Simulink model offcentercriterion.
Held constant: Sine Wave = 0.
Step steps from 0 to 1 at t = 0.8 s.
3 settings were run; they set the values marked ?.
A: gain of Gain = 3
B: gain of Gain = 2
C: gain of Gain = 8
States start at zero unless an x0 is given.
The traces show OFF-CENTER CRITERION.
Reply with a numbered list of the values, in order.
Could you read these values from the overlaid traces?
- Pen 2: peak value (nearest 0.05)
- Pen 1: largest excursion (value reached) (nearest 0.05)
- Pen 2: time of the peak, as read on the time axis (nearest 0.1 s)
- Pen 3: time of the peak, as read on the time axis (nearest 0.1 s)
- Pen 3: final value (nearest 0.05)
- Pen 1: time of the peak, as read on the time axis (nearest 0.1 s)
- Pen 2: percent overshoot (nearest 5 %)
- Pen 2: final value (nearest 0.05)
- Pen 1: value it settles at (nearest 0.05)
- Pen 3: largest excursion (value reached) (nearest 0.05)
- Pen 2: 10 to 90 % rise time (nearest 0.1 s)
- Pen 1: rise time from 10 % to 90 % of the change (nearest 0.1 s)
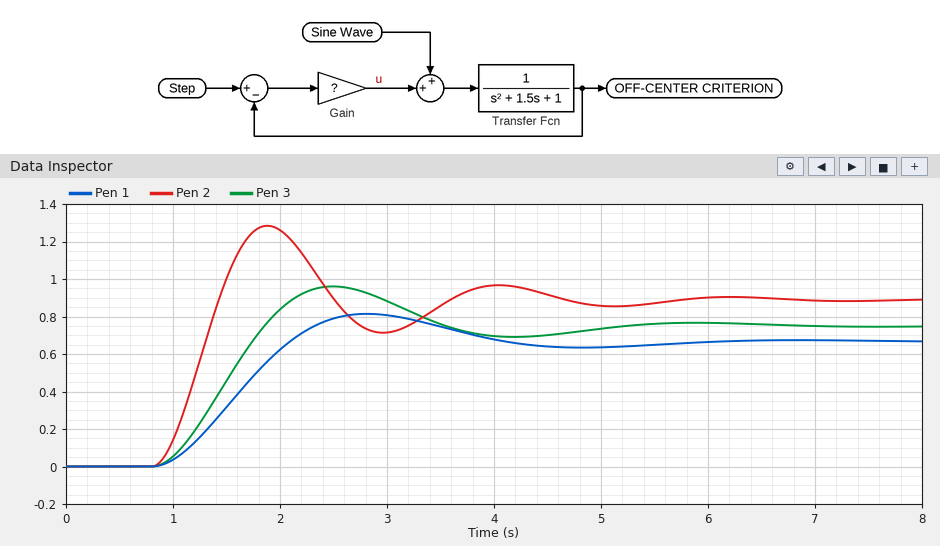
1. 1.30
2. 0.80
3. 1.9 s
4. 2.5 s
5. 0.75
6. 2.8 s
7. 45 %
8. 0.90
9. 0.65
10. 0.95
11. 0.4 s
12. 0.9 s
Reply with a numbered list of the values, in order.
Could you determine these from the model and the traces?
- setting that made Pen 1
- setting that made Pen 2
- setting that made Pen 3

1. B
2. C
3. A
